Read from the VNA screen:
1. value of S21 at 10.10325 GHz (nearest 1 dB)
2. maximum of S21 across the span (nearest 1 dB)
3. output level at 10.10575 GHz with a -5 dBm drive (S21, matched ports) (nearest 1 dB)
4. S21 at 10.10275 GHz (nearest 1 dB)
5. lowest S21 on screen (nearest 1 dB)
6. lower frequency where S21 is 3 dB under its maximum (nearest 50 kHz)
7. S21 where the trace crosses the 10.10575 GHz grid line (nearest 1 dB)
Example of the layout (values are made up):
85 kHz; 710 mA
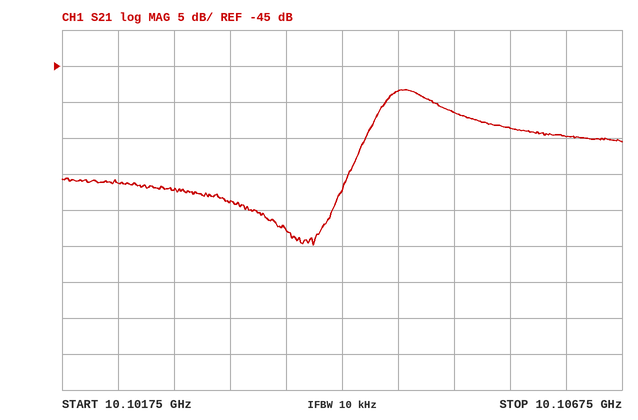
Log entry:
-64 dB; -48 dB; -59 dBm; -62 dB; -70 dB; 10.10460 GHz; -54 dB
